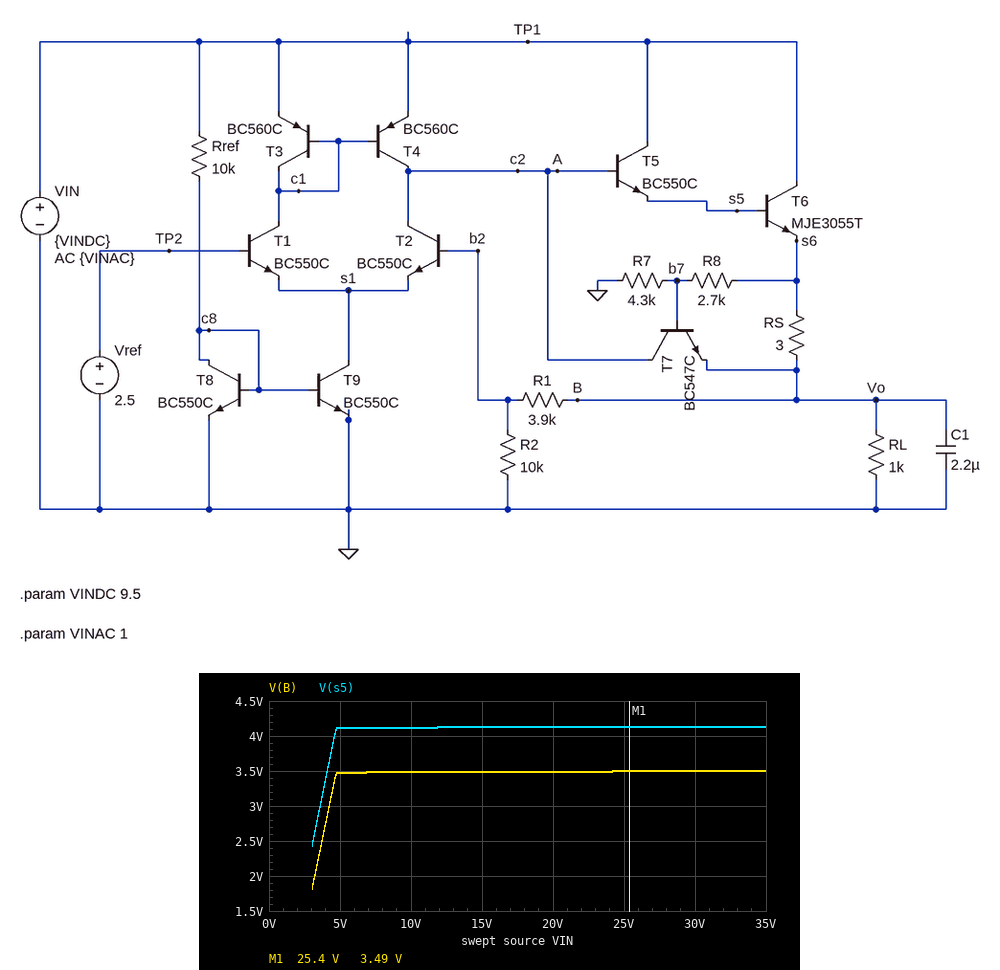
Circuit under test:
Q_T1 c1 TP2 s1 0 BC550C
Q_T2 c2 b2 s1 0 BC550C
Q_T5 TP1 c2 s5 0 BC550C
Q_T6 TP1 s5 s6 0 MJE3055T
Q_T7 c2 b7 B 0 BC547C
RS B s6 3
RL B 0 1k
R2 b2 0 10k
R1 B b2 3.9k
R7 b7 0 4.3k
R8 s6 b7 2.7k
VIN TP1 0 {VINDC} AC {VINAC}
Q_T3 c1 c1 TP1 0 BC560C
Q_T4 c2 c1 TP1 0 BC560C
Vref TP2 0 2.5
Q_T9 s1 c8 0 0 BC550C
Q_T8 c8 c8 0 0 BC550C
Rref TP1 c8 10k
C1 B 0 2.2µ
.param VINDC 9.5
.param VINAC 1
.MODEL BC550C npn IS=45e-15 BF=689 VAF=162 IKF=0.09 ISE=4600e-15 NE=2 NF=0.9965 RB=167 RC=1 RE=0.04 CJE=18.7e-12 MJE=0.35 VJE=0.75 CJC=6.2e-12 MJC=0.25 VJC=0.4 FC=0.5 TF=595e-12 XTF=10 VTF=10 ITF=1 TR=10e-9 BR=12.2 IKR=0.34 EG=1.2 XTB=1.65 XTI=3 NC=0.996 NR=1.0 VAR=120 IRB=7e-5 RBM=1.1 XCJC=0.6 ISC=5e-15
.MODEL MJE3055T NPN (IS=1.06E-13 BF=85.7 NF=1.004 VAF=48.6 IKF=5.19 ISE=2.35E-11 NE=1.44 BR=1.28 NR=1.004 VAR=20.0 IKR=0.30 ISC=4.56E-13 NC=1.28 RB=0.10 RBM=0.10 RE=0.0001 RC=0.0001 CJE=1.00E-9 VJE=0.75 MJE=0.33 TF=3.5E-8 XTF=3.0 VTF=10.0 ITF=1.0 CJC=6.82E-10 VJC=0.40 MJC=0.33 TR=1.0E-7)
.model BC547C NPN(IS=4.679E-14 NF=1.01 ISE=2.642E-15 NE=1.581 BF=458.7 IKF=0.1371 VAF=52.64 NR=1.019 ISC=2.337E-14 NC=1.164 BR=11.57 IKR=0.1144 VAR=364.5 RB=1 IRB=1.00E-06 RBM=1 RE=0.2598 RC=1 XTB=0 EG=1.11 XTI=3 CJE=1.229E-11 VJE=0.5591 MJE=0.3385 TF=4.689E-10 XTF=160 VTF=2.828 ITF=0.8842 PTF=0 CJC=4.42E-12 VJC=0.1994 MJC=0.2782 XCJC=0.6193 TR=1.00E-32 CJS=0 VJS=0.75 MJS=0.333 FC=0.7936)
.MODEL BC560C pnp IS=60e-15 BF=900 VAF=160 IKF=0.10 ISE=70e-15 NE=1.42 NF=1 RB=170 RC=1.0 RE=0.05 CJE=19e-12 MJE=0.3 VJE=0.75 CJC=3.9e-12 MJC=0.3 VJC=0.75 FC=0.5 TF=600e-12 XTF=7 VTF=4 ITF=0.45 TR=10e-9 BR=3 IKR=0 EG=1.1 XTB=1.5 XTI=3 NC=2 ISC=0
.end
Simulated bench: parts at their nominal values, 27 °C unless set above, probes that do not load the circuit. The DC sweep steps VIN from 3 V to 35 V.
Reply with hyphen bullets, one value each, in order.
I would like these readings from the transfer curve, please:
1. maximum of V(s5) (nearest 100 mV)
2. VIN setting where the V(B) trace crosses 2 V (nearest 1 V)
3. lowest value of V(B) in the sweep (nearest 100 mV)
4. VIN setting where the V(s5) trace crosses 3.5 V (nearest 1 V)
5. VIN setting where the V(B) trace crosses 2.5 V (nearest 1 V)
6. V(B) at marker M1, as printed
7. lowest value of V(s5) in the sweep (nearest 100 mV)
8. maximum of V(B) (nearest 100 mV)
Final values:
- 4.1 V
- 3 V
- 1.8 V
- 4 V
- 4 V
- 3.49 V
- 2.4 V
- 3.5 V
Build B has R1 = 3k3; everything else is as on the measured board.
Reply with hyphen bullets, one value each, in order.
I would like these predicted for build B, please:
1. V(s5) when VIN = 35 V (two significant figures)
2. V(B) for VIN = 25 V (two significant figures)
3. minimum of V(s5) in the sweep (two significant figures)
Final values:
- 4.0 V
- 3.3 V
- 2.4 V
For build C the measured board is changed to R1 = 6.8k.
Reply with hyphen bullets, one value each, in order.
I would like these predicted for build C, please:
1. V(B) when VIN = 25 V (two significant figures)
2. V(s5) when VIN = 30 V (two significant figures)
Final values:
- 4.2 V
- 4.9 V
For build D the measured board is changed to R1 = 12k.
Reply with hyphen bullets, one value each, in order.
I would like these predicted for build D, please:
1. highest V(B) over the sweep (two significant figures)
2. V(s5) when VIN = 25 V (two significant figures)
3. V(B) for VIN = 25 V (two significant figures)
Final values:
- 5.6 V
- 6.2 V
- 5.5 V
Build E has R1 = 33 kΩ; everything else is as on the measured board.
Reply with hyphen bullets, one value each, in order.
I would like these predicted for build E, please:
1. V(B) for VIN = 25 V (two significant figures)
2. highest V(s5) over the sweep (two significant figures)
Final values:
- 11 V
- 12 V
